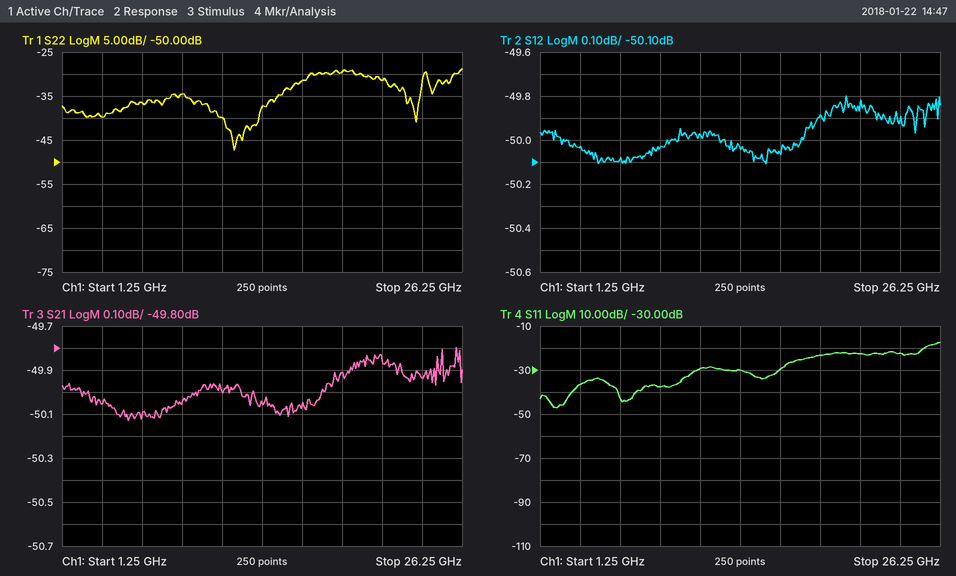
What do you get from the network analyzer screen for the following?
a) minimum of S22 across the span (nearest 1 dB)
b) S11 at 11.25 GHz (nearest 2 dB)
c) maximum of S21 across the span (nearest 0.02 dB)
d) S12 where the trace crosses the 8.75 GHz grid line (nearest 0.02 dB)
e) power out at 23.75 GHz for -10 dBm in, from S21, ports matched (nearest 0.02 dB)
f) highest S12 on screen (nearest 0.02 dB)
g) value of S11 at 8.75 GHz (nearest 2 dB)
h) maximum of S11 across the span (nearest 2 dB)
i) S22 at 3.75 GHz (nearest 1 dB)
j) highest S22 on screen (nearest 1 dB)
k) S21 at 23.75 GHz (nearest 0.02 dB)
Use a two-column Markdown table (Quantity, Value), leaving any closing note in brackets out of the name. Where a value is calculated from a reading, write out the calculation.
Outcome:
| Quantity | Value |
|---|---|
| minimum of S22 across the span | -47 dB |
| S11 at 11.25 GHz | -30 dB |
| maximum of S21 across the span | -49.80 dB |
| S12 where the trace crosses the 8.75 GHz grid line | -50.04 dB |
| power out at 23.75 GHz for -10 dBm in, from S21, ports matched | -10 dBm + (-49.94 dB) = -59.94 dBm |
| highest S12 on screen | -49.80 dB |
| value of S11 at 8.75 GHz | -38 dB |
| maximum of S11 across the span | -18 dB |
| S22 at 3.75 GHz | -40 dB |
| highest S22 on screen | -29 dB |
| S21 at 23.75 GHz | -49.94 dB |
